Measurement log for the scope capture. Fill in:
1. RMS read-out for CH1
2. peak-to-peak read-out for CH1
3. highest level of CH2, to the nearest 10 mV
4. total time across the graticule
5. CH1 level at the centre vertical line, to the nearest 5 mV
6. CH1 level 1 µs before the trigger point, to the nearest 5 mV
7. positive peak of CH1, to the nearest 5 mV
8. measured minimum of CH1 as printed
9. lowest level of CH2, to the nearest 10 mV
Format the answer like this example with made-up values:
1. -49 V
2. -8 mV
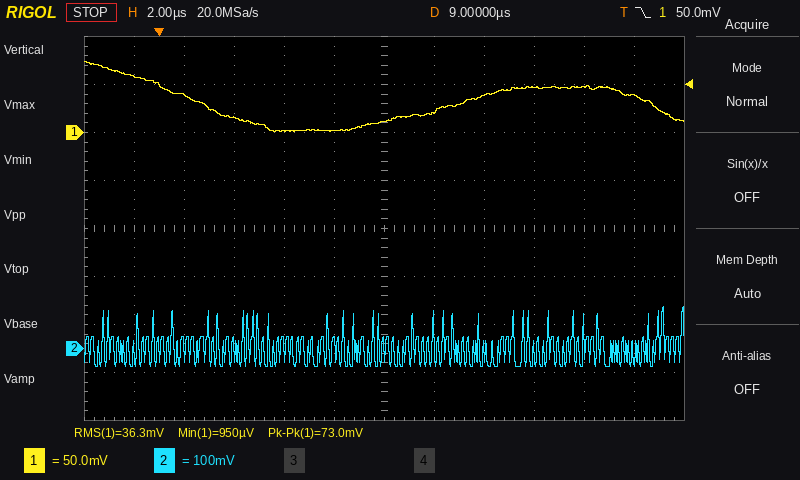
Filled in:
1. 36.3 mV
2. 73.0 mV
3. 90 mV
4. 24 µs
5. 10 mV
6. 60 mV
7. 75 mV
8. 950 µV
9. -40 mV
